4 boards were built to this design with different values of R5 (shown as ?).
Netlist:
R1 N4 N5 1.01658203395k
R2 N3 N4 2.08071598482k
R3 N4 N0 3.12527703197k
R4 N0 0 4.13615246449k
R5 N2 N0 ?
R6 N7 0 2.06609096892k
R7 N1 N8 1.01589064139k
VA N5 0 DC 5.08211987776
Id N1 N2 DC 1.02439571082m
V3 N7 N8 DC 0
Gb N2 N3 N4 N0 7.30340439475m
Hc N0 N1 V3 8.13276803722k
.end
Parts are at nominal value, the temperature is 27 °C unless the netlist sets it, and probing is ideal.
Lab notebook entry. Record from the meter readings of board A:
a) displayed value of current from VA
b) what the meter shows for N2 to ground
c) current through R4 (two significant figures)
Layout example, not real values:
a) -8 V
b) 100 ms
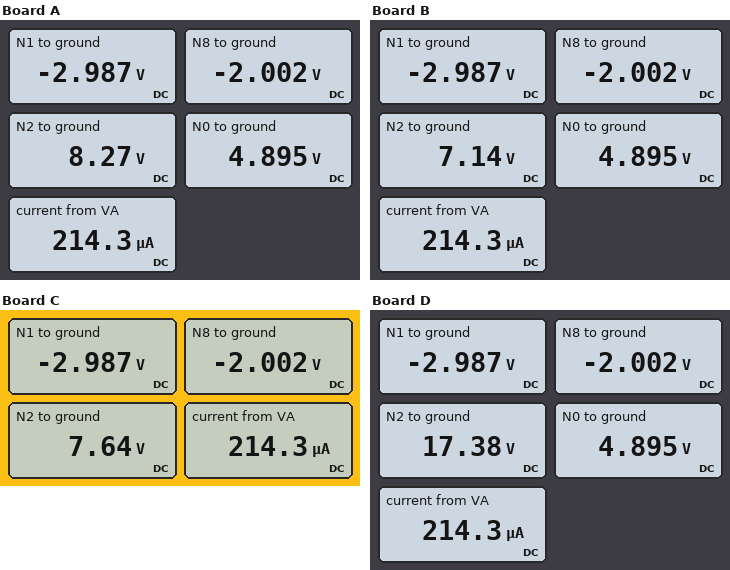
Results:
a) 214.3 µA
b) 8.27 V
c) 1.2 mA
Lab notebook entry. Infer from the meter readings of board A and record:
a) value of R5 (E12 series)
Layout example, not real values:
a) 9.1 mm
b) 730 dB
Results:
a) 2.7 kΩ
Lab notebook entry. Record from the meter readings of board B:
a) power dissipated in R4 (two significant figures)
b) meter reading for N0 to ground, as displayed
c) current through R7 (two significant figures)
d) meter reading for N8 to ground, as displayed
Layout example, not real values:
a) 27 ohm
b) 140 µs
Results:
a) 5.8 mW
b) 4.895 V
c) 970 µA
d) -2.002 V
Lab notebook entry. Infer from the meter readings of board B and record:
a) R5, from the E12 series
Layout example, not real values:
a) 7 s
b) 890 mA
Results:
a) 1.8 kΩ
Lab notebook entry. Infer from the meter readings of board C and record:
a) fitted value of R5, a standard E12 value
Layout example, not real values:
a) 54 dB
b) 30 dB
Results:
a) 2.2 kΩ
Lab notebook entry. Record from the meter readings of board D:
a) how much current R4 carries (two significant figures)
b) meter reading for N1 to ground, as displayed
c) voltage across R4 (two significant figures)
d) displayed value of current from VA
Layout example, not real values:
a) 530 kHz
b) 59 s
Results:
a) 1.2 mA
b) -2.987 V
c) 4.9 V
d) 214.3 µA
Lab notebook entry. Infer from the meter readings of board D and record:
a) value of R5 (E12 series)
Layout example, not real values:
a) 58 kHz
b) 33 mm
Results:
a) 10 kΩ
